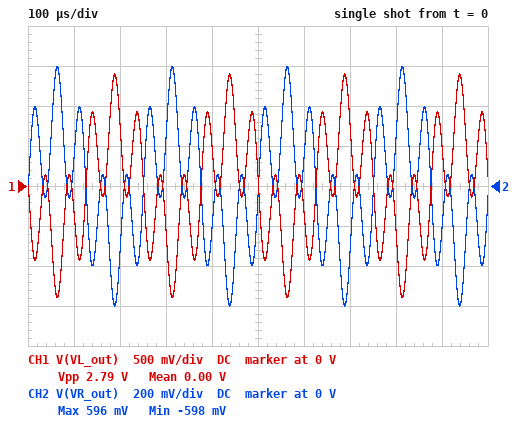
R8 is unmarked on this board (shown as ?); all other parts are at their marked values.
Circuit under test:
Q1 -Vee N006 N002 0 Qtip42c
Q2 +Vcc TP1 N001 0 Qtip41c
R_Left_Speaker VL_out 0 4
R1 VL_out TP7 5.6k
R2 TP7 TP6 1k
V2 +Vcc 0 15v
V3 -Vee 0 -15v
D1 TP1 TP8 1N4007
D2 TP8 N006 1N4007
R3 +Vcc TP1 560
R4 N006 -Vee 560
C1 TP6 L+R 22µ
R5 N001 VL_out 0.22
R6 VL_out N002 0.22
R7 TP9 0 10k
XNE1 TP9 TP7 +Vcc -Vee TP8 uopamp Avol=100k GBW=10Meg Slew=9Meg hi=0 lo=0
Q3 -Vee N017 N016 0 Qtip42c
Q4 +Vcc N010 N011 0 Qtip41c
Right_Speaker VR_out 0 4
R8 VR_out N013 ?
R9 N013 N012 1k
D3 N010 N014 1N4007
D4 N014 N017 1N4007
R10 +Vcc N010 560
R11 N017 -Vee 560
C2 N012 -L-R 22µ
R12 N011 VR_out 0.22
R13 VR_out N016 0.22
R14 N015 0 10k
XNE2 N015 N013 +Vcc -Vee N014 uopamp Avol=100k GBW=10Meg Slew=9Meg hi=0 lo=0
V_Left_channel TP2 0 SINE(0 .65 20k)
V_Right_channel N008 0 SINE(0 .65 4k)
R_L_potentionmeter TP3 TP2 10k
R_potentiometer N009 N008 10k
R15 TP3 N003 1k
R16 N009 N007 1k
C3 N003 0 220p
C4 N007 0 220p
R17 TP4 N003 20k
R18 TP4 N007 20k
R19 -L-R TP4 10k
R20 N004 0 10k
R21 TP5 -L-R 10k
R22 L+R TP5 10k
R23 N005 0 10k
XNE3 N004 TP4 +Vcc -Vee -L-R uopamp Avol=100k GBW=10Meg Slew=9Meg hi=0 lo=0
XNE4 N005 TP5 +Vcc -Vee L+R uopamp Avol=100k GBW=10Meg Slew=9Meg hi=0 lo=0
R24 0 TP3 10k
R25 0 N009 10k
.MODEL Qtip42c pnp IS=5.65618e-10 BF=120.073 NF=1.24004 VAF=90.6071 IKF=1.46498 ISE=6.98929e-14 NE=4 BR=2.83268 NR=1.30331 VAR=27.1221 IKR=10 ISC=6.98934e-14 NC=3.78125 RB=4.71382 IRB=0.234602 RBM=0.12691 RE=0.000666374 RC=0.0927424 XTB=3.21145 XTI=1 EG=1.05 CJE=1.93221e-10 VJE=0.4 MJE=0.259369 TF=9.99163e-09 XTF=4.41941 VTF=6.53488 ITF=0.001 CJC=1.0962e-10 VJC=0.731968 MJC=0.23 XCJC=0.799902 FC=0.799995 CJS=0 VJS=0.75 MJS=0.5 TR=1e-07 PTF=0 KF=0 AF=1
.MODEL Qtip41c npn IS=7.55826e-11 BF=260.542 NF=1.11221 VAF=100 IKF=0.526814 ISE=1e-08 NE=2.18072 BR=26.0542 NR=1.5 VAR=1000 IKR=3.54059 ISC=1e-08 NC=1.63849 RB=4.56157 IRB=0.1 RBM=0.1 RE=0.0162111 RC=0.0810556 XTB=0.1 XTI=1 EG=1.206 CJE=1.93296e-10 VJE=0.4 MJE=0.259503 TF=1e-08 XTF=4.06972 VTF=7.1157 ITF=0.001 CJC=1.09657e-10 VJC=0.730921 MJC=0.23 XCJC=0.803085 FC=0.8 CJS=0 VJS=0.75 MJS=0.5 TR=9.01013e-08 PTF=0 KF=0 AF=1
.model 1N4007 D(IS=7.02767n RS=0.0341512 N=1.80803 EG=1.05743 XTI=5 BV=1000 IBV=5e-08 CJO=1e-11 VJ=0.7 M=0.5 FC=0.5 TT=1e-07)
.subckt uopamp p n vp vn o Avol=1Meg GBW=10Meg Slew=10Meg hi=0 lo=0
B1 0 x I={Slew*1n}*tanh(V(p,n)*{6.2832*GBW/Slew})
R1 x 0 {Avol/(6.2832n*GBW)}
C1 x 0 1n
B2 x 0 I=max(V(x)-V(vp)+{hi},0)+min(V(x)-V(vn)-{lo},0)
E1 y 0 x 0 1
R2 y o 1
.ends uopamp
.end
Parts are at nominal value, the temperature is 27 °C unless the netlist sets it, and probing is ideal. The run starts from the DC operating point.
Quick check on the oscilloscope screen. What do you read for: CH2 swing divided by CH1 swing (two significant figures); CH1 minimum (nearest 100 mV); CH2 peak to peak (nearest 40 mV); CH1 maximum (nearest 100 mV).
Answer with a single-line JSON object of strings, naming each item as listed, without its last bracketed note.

{"CH2 swing divided by CH1 swing": "0.43", "CH1 minimum": "-1.4 V", "CH2 peak to peak": "1.20 V", "CH1 maximum": "1.4 V"}
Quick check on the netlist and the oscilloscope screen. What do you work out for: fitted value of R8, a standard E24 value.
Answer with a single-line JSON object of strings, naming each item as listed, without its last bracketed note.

{"fitted value of R8, a standard E24 value": "2.4 kΩ"}
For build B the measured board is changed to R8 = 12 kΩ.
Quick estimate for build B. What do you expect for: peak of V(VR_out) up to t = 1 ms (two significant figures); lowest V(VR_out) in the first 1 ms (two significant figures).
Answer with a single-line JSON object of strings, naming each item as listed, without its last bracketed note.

{"peak of V(VR_out) up to t = 1 ms": "3.0 V", "lowest V(VR_out) in the first 1 ms": "-3.0 V"}
